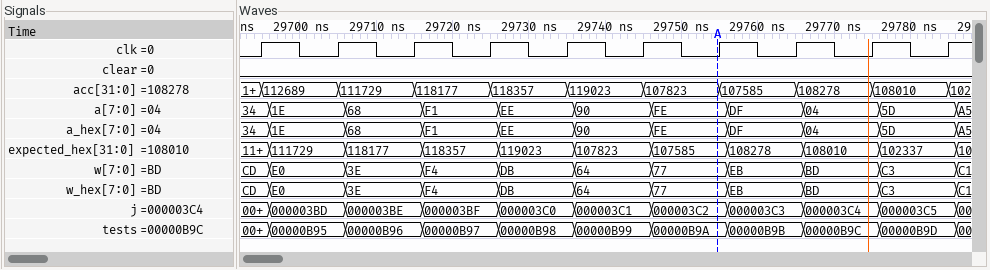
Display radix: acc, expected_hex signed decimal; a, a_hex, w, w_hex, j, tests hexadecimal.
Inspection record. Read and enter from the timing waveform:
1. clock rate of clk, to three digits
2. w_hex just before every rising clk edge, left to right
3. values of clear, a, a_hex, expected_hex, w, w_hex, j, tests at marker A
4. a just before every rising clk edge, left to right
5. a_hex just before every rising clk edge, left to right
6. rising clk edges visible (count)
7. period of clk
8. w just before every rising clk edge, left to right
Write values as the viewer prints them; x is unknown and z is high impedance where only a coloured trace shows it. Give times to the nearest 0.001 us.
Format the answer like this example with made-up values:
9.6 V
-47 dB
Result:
100 MHz
CD, E0, 3E, F4, DB, 64, 77, EB, BD, C3
clear=0, a=FE, a_hex=FE, expected_hex=107585, w=77, w_hex=77, j=000003C2, tests=00000B9A
34, 1E, 68, F1, EE, 90, FE, DF, 04, 5D
34, 1E, 68, F1, EE, 90, FE, DF, 04, 5D
10
0.01 us
CD, E0, 3E, F4, DB, 64, 77, EB, BD, C3
